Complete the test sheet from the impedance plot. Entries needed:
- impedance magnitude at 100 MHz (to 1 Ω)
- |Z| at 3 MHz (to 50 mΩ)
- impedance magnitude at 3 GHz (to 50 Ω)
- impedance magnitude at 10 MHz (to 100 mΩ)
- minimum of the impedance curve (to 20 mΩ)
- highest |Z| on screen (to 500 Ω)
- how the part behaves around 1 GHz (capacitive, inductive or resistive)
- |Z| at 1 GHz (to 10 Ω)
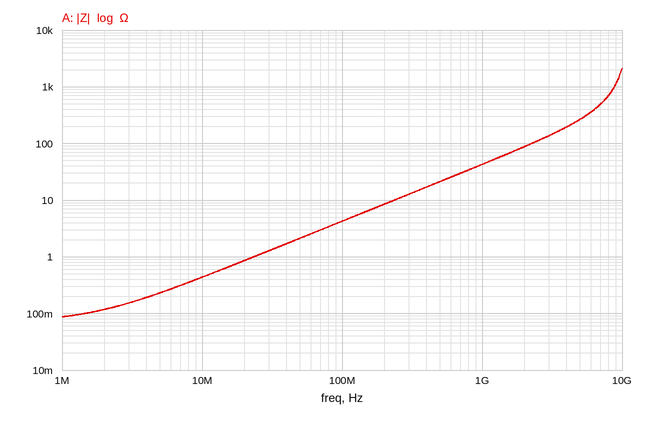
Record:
4 Ω
150 mΩ
150 Ω
400 mΩ
80 mΩ
2.0 kΩ
inductive
40 Ω
